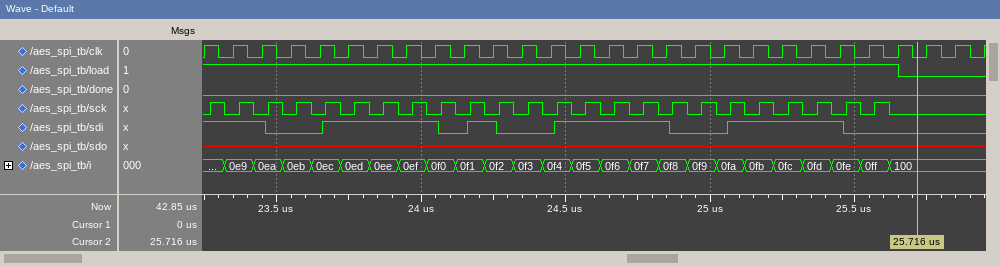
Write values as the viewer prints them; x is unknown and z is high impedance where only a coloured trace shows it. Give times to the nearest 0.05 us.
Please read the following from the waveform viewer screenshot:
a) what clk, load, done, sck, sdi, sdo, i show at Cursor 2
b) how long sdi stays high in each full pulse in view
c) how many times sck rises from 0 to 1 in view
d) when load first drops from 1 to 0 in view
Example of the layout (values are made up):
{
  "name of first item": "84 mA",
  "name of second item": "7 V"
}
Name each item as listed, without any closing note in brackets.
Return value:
{
  "what clk, load, done, sck, sdi, sdo, i show at Cursor 2": "clk=0, load=0, done=0, sck=0, sdi=0, sdo=x, i=100",
  "how long sdi stays high in each full pulse in view": "0.4 us, 0.1 us, 0.4 us, 0.4 us",
  "how many times sck rises from 0 to 1 in view": "24",
  "when load first drops from 1 to 0 in view": "25.65 us"
}
